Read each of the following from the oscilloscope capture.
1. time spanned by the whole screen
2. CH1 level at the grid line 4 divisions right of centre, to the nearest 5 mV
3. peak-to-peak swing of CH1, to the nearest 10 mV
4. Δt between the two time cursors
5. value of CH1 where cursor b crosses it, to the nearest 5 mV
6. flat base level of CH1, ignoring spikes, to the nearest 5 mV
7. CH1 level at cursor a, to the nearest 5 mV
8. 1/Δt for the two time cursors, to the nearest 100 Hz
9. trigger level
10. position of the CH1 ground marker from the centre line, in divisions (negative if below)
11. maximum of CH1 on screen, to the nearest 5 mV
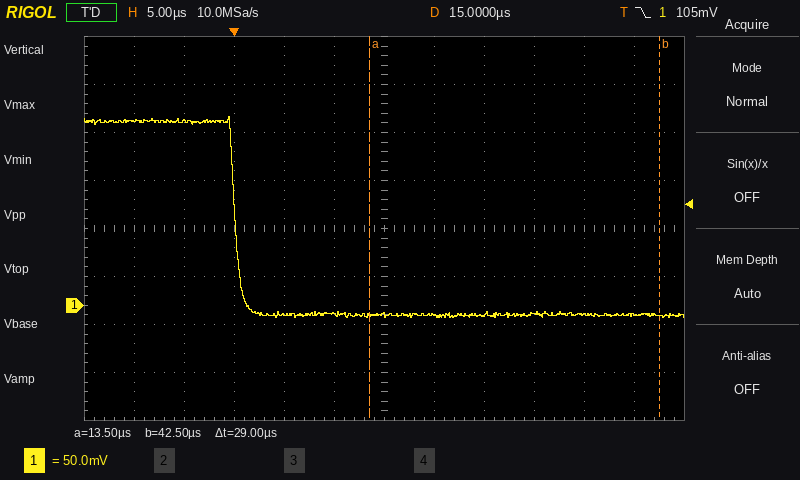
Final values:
60 µs
-10 mV
210 mV
29 µs
-10 mV
-10 mV
-10 mV
34.5 kHz
105 mV
-1.6 div
195 mV
